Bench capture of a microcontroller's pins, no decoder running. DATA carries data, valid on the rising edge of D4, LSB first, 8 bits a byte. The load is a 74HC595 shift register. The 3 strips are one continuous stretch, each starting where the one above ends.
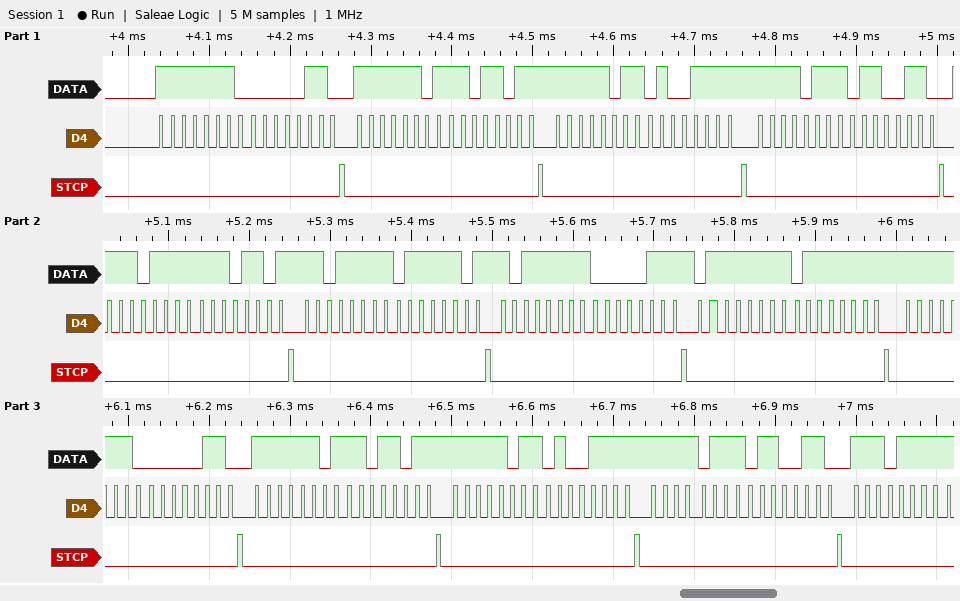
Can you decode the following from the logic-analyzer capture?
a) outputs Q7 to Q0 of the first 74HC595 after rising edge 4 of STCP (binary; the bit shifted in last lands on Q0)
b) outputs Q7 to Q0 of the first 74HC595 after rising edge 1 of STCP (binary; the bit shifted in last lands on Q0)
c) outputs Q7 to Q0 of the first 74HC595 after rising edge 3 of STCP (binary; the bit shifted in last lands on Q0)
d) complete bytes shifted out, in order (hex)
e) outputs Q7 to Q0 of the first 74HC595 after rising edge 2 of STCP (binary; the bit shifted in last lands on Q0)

01100110
00000110
01001111
7F 60 BF DB DF F2 EF 66 F7 B7 FB BE FD E0 FE FE 7F 60 BF DB DF F2 EF 66 F7
11011011
